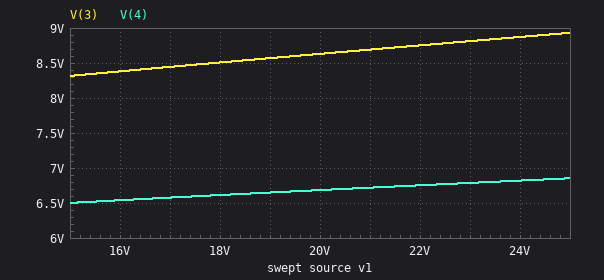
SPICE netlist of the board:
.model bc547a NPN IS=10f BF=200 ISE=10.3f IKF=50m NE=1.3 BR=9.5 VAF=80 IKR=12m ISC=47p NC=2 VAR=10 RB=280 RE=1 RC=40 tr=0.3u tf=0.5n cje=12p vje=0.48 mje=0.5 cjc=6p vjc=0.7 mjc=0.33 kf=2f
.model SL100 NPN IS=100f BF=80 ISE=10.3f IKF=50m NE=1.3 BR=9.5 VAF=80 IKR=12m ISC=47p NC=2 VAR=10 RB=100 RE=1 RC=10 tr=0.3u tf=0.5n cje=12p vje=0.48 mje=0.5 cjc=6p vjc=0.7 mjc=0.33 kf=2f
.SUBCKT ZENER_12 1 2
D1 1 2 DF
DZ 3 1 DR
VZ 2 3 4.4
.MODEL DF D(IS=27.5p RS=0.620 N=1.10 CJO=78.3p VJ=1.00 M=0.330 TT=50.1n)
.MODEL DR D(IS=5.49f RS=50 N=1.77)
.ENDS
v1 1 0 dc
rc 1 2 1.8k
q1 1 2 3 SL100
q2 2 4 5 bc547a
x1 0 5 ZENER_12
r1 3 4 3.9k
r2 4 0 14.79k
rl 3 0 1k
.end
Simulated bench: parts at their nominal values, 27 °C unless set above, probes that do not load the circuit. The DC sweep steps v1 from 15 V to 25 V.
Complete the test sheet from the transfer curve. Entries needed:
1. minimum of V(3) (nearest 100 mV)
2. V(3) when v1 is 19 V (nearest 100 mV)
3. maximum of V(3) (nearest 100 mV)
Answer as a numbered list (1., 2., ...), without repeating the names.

1. 8.3 V
2. 8.6 V
3. 8.9 V
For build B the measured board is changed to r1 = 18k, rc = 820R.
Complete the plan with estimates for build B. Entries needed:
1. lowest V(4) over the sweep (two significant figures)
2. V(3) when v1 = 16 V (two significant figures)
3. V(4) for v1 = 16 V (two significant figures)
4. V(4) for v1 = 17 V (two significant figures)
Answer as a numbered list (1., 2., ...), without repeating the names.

1. 6.2 V
2. 14 V
3. 6.3 V
4. 6.4 V
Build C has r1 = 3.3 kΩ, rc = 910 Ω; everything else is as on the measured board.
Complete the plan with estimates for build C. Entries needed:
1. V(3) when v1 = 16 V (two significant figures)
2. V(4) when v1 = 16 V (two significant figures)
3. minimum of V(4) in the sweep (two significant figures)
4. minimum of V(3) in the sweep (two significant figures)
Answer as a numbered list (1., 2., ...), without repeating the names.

1. 8.5 V
2. 6.8 V
3. 6.7 V
4. 8.4 V
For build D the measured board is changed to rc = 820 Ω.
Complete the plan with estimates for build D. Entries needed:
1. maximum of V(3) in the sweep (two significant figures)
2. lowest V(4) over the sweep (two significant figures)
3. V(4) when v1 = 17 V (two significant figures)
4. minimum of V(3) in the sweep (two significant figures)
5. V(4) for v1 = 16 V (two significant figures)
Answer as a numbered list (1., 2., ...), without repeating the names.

1. 10 V
2. 6.7 V
3. 6.9 V
4. 8.7 V
5. 6.8 V
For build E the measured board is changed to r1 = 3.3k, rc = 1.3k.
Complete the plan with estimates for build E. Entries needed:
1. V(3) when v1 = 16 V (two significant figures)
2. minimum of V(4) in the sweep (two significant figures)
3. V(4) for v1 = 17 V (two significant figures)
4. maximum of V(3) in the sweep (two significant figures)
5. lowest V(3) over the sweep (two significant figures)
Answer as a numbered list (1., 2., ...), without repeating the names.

1. 8.3 V
2. 6.6 V
3. 6.7 V
4. 9.0 V
5. 8.2 V
